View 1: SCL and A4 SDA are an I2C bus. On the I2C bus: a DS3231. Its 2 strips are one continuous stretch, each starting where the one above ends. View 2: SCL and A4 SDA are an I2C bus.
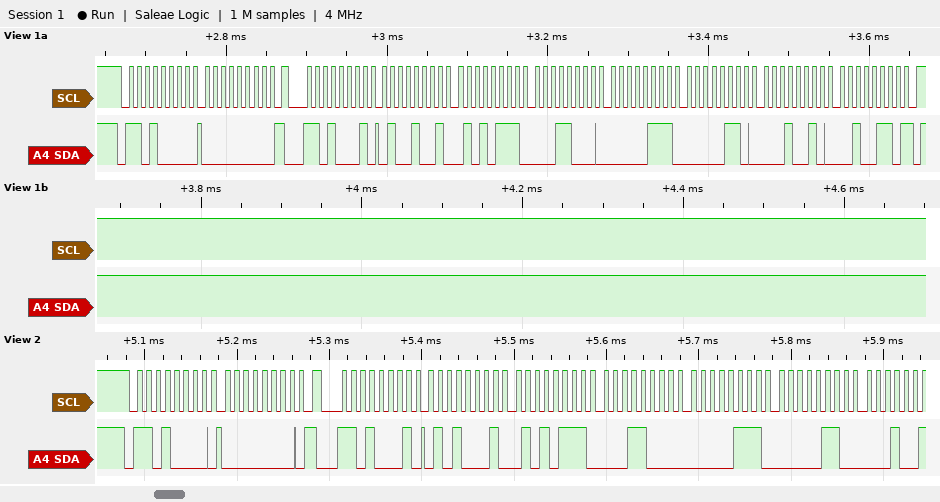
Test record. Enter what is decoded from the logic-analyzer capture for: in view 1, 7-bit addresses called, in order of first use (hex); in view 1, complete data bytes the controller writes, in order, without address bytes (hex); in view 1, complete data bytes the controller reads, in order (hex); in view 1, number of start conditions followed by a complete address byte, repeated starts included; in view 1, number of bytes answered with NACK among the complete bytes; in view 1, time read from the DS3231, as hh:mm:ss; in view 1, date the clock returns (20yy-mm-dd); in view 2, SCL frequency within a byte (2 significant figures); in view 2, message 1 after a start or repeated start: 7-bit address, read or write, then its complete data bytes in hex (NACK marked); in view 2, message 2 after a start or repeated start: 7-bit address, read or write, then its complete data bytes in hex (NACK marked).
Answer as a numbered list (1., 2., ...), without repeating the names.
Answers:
1. 0x68
2. 00
3. 49 57 18 07 06 12 26
4. 2
5. 1
6. 18:57:49
7. 2026-12-06
8. 100 kHz
9. 0x68 write: 00
10. 0x68 read: 51 57 18 07 06
